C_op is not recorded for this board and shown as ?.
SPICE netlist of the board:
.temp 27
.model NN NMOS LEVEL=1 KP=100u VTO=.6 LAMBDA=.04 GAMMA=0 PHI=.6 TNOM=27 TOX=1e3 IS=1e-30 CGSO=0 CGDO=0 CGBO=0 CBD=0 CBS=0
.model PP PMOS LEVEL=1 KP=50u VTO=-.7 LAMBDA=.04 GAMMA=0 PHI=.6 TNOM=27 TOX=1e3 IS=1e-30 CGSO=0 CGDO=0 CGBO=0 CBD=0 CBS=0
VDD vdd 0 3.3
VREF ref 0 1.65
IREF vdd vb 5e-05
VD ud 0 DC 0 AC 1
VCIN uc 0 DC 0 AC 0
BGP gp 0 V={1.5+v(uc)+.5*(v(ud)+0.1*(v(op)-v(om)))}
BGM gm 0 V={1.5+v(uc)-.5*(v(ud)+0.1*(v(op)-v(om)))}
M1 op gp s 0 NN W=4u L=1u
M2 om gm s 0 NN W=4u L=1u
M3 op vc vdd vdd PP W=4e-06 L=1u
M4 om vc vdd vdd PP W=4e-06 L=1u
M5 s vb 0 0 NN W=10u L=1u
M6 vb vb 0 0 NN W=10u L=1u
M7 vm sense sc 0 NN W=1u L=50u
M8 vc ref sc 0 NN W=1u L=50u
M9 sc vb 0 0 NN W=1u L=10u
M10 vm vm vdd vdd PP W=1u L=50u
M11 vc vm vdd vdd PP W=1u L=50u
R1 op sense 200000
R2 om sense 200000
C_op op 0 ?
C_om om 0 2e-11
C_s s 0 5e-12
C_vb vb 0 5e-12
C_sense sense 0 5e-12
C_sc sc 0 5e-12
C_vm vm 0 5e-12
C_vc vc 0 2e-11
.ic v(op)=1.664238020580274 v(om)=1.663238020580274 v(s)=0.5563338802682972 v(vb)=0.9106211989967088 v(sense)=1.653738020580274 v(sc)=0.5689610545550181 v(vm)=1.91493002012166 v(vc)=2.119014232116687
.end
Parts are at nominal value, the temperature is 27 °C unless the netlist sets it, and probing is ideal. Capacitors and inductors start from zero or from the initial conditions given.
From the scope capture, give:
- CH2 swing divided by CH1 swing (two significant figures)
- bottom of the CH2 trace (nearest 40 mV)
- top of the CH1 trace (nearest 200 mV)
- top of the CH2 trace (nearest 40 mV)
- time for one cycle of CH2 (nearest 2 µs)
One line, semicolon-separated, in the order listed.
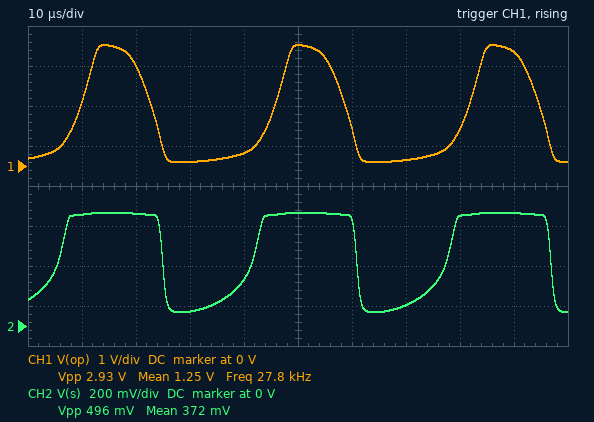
0.17; 80 mV; 3.0 V; 560 mV; 36 µs
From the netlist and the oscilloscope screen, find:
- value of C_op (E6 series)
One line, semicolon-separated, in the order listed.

33 pF
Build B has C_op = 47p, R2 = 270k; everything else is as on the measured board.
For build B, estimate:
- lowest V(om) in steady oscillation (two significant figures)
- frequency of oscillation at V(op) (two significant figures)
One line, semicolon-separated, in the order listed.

90 mV; 26 kHz
